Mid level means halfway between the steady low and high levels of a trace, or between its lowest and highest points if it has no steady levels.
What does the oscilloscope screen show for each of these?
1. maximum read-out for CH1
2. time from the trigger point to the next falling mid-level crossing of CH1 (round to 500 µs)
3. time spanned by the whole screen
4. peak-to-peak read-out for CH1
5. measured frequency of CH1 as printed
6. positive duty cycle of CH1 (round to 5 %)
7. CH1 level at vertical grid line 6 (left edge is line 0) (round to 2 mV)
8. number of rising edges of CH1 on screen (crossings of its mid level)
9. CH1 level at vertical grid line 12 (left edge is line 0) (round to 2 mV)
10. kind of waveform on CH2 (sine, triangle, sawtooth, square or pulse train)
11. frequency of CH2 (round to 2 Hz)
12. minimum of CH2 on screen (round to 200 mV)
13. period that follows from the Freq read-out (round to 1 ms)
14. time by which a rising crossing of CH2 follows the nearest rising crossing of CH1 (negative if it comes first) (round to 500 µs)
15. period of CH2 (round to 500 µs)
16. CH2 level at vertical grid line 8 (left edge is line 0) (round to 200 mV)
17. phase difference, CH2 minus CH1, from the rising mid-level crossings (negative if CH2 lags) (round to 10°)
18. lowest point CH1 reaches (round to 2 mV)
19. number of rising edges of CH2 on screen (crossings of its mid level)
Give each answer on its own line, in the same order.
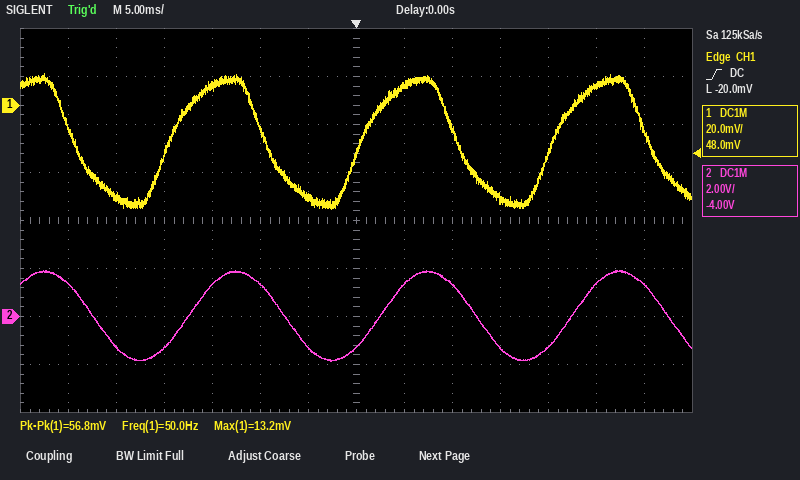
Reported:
13.2 mV
10.5 ms
70 ms
56.8 mV
50.0 Hz
50 %
-38 mV
3
8 mV
sine
50 Hz
-1.8 V
20 ms
+2.0 ms
20.0 ms
1.4 V
-40°
-44 mV
3
